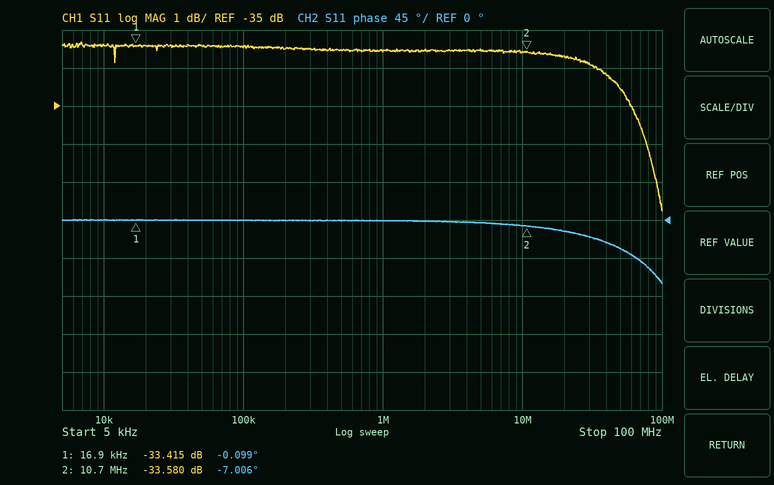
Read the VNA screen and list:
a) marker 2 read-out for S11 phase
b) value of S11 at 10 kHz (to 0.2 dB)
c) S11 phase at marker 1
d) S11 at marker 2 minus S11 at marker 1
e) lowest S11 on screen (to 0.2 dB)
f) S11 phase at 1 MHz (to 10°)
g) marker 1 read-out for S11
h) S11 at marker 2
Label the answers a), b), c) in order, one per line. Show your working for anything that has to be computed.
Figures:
a) -7.006°
b) -33.4 dB
c) -0.099°
d) -33.58 − (-33.415) = -0.165 dB
e) -37.8 dB
f) 0°
g) -33.415 dB
h) -33.580 dB
